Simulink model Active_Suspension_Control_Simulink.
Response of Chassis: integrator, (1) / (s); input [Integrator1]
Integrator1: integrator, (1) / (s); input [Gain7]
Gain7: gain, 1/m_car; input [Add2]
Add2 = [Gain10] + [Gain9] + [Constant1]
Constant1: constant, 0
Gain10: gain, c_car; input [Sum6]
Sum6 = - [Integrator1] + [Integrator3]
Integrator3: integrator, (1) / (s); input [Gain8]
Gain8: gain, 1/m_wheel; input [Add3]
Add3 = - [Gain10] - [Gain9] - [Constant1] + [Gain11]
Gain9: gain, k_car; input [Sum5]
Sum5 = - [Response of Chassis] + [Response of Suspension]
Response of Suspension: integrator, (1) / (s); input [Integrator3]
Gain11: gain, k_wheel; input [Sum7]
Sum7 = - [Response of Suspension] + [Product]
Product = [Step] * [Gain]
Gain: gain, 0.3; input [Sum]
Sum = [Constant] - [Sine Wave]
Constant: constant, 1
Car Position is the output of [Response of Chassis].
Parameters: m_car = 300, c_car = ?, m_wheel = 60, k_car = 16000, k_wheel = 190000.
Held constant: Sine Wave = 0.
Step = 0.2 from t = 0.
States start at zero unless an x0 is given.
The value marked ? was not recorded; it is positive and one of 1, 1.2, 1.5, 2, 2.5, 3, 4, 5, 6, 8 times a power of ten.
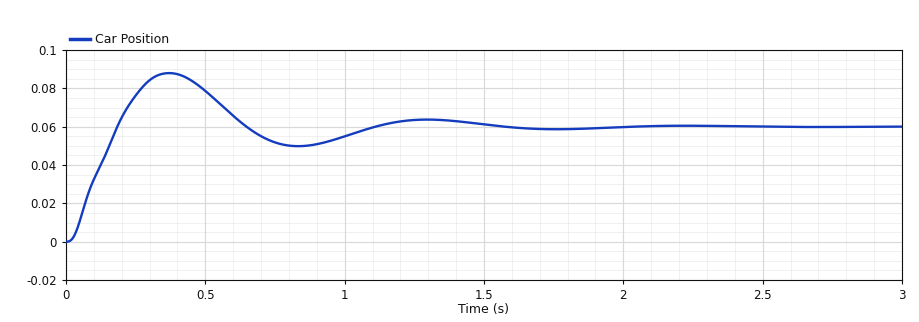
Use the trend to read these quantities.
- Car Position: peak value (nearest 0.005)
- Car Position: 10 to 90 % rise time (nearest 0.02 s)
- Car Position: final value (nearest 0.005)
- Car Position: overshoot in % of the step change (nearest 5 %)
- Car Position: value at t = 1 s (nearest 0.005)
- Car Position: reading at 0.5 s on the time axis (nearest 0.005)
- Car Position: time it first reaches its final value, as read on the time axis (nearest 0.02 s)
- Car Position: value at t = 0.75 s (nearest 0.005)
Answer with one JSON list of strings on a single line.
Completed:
["0.090", "0.12 s", "0.060", "45 %", "0.055", "0.080", "0.18 s", "0.050"]
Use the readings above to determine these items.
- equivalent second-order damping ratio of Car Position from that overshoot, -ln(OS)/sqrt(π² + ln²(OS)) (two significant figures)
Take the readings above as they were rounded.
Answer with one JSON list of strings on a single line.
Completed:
["0.25"]
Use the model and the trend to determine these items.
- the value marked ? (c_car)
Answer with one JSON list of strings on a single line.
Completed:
["1500"]
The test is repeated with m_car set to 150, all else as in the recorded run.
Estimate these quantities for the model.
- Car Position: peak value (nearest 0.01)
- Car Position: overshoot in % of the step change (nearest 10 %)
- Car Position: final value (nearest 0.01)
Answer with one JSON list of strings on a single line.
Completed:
["0.08", "40 %", "0.06"]
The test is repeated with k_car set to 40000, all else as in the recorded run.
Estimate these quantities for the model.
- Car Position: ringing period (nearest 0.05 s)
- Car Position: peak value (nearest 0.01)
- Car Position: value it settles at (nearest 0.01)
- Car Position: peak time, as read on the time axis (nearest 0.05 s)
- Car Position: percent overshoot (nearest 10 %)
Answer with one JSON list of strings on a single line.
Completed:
["0.60 s", "0.10", "0.06", "0.25 s", "70 %"]
